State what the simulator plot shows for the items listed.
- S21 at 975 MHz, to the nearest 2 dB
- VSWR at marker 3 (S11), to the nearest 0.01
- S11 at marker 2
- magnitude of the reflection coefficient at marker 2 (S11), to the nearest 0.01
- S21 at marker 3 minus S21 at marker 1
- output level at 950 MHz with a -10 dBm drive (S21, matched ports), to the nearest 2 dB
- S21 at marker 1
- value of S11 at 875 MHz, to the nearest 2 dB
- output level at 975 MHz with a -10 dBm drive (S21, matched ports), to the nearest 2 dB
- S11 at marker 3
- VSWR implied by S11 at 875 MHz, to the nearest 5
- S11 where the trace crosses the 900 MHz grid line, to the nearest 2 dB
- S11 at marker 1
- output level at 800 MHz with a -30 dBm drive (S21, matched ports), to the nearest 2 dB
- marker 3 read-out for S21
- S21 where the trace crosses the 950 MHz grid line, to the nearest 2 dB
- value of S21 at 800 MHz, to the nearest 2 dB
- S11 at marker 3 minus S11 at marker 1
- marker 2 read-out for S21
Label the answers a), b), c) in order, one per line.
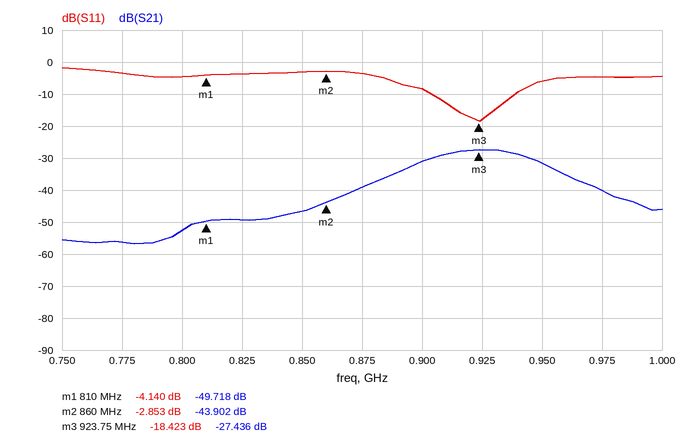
a) -40 dB
b) 1.27
c) -2.853 dB
d) 0.72
e) 22.282 dB
f) -42 dBm
g) -49.718 dB
h) -4 dB
i) -50 dBm
j) -18.423 dB
k) 5
l) -8 dB
m) -4.140 dB
n) -82 dBm
o) -27.436 dB
p) -32 dB
q) -52 dB
r) -14.283 dB
s) -43.902 dB
